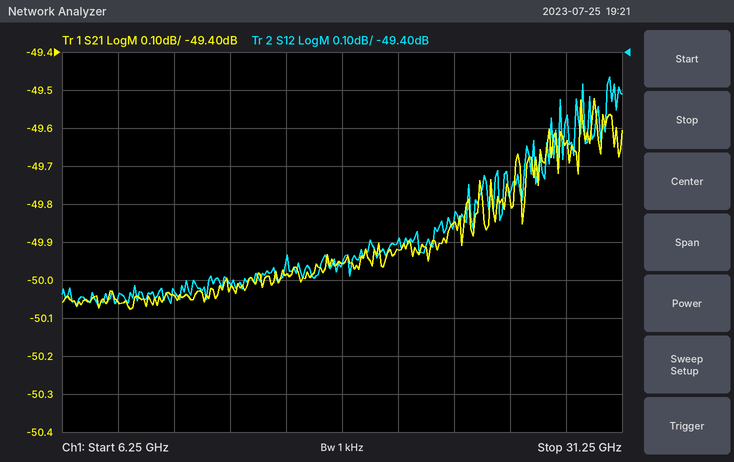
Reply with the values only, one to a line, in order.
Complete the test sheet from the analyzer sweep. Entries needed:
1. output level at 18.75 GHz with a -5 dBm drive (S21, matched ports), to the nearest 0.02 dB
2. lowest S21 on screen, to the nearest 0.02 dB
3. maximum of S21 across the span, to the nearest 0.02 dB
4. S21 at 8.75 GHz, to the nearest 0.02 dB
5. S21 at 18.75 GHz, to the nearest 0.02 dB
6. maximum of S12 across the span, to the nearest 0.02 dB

-54.96 dBm
-50.08 dB
-49.52 dB
-50.06 dB
-49.96 dB
-49.46 dB
